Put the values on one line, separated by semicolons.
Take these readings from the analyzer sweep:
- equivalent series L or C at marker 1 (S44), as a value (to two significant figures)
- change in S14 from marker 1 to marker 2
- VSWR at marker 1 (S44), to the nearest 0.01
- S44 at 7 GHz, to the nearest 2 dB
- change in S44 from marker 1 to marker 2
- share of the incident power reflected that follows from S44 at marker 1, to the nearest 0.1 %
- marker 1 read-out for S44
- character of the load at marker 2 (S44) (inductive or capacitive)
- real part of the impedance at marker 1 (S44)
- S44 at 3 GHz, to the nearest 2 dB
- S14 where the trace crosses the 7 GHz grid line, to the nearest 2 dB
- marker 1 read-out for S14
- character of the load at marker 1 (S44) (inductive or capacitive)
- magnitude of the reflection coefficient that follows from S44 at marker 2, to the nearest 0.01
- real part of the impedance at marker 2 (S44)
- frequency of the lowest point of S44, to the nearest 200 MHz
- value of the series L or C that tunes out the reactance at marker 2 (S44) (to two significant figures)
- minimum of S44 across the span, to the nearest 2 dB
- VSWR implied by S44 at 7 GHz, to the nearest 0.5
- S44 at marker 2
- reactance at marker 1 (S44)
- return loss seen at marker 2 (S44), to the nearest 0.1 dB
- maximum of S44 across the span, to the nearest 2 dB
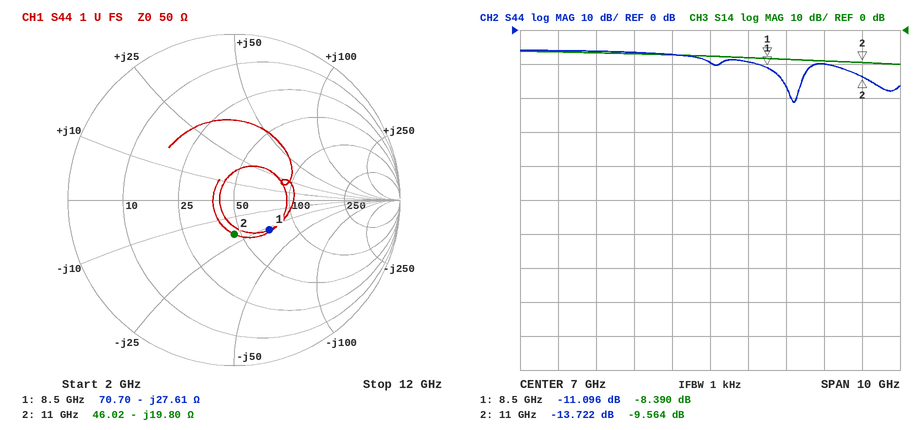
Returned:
680 fF; -1.174 dB; 1.77; -10 dB; -2.626 dB; 7.8 %; -11.096 dB; capacitive; 70.70 Ω; -6 dB; -8 dB; -8.390 dB; capacitive; 0.21; 46.02 Ω; 9.2 GHz; 290 pH; -22 dB; 2.0; -13.722 dB; -27.61 Ω; 13.7 dB; -6 dB
